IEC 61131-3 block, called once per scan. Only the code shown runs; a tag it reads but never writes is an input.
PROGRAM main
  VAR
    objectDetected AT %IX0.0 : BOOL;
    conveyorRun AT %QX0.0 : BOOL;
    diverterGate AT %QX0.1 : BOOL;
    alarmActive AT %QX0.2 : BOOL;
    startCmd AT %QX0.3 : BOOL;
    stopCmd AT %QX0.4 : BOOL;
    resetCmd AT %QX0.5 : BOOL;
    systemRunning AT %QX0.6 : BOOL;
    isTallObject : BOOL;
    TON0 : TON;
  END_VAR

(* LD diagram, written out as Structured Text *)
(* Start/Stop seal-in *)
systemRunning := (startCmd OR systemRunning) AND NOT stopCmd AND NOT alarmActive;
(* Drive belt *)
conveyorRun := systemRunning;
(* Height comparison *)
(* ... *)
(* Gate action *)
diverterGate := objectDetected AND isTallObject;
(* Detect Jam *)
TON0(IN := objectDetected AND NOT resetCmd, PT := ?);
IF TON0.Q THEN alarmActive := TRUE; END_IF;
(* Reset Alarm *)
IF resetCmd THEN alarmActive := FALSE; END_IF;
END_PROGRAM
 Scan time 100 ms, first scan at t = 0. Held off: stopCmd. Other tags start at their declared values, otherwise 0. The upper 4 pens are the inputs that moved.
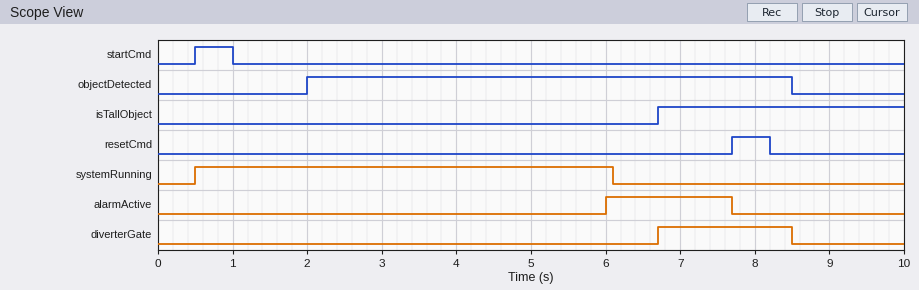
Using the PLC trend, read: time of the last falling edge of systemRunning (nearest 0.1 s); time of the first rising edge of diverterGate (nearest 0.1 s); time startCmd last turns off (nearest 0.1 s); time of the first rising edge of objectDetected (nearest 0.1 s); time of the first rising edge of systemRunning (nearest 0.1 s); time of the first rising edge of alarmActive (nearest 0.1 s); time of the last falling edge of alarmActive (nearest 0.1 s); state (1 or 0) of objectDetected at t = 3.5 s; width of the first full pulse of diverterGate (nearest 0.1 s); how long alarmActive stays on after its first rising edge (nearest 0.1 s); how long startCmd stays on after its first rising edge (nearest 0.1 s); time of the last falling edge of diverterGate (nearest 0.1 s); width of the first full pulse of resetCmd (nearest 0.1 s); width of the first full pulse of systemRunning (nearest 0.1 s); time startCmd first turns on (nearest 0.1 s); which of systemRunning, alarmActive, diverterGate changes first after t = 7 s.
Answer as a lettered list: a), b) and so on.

a) 6.1 s
b) 6.7 s
c) 1.0 s
d) 2.0 s
e) 0.5 s
f) 6.0 s
g) 7.7 s
h) 1
i) 1.8 s
j) 1.7 s
k) 0.5 s
l) 8.5 s
m) 0.5 s
n) 5.6 s
o) 0.5 s
p) alarmActive
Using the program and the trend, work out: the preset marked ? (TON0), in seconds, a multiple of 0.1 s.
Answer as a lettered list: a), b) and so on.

a) 4.0 s
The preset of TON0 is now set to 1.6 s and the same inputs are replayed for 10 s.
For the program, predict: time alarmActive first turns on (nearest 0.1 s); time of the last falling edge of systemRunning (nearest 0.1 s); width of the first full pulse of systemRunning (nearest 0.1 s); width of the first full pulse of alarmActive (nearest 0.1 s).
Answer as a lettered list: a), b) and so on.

a) 3.6 s
b) 3.7 s
c) 3.2 s
d) 4.1 s
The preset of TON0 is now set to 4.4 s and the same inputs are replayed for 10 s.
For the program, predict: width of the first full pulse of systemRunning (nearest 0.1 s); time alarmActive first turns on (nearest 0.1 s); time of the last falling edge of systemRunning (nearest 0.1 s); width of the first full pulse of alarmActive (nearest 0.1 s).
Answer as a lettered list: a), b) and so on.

a) 6.0 s
b) 6.4 s
c) 6.5 s
d) 1.3 s
